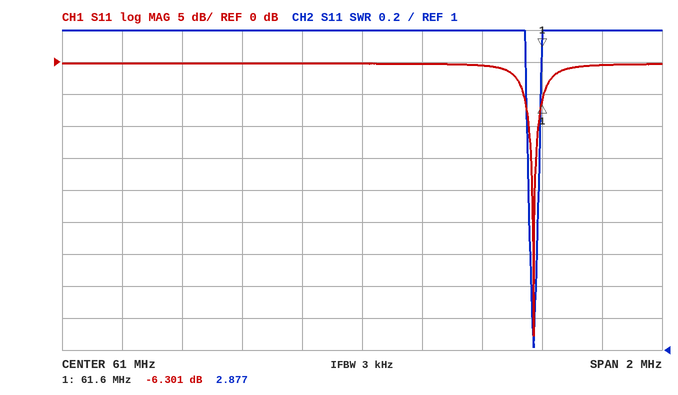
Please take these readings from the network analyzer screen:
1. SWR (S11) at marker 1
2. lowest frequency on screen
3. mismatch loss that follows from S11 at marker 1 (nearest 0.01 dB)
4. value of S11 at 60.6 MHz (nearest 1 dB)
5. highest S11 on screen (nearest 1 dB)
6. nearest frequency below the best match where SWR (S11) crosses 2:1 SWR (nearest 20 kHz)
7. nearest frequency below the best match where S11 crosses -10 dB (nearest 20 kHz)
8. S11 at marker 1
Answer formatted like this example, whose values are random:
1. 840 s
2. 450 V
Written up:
1. 2.877
2. 60 MHz
3. 1.16 dB
4. 0 dB
5. 0 dB
6. 61.56 MHz
7. 61.56 MHz
8. -6.301 dB
